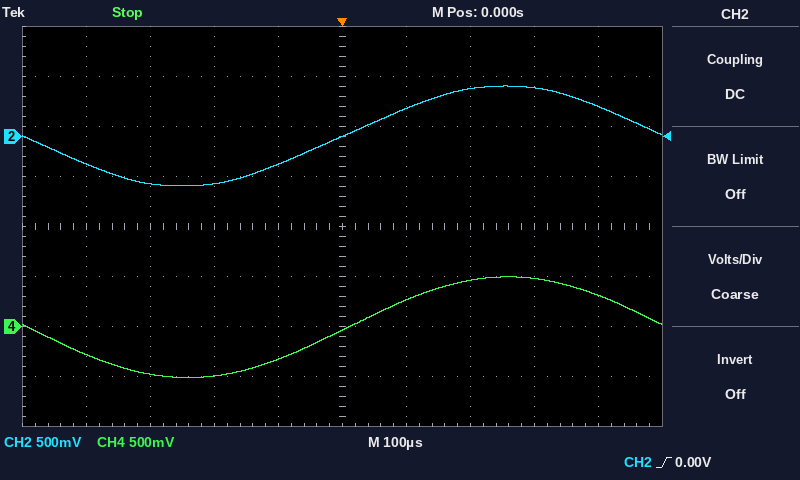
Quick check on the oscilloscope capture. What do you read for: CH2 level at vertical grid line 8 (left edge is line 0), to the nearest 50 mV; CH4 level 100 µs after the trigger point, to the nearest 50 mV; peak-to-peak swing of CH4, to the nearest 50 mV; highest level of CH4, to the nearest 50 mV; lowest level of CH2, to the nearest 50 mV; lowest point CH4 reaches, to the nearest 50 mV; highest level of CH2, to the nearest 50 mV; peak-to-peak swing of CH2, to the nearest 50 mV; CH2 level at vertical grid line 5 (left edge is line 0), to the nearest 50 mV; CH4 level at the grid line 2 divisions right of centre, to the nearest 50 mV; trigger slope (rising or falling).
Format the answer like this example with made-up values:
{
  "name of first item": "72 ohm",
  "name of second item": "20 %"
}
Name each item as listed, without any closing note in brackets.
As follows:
{
  "CH2 level at vertical grid line 8 (left edge is line 0), to the nearest 50 mV": "500 mV",
  "CH4 level 100 µs after the trigger point, to the nearest 50 mV": "250 mV",
  "peak-to-peak swing of CH4, to the nearest 50 mV": "1.00 V",
  "highest level of CH4, to the nearest 50 mV": "500 mV",
  "lowest level of CH2, to the nearest 50 mV": "-500 mV",
  "lowest point CH4 reaches, to the nearest 50 mV": "-500 mV",
  "highest level of CH2, to the nearest 50 mV": "500 mV",
  "peak-to-peak swing of CH2, to the nearest 50 mV": "1.00 V",
  "CH2 level at vertical grid line 5 (left edge is line 0), to the nearest 50 mV": "0 mV",
  "CH4 level at the grid line 2 divisions right of centre, to the nearest 50 mV": "450 mV",
  "trigger slope": "rising"
}
